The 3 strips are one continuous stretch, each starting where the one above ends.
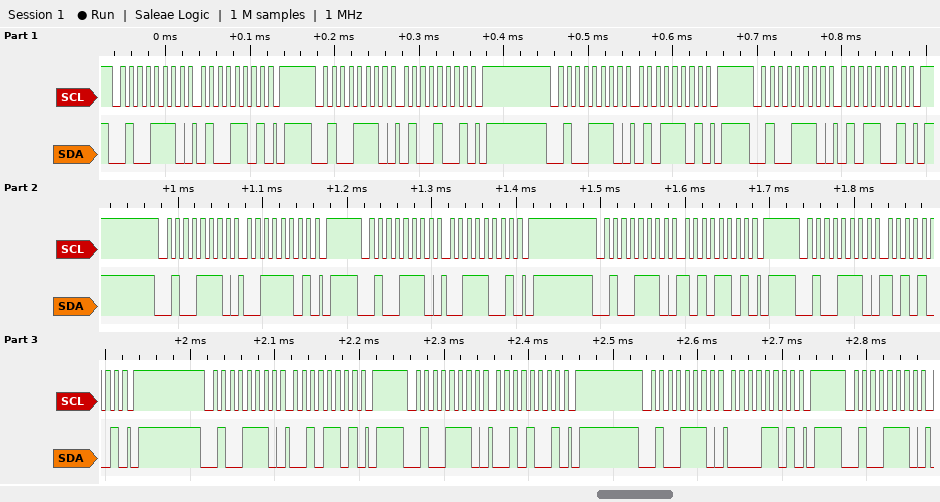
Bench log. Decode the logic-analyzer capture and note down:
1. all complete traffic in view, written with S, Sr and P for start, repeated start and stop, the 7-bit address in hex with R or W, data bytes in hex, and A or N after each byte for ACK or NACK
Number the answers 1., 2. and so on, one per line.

1. S 27W A 4D A P S 27W A 49 A P S 27W A 5D A P S 27W A 59 A P S 27W A 3D A P S 27W A 39 A P S 27W A AD A P S 27W A A9 A P S 27W A 2D A P S 27W A 29 A P S 27W A 0D A P S 27W A
